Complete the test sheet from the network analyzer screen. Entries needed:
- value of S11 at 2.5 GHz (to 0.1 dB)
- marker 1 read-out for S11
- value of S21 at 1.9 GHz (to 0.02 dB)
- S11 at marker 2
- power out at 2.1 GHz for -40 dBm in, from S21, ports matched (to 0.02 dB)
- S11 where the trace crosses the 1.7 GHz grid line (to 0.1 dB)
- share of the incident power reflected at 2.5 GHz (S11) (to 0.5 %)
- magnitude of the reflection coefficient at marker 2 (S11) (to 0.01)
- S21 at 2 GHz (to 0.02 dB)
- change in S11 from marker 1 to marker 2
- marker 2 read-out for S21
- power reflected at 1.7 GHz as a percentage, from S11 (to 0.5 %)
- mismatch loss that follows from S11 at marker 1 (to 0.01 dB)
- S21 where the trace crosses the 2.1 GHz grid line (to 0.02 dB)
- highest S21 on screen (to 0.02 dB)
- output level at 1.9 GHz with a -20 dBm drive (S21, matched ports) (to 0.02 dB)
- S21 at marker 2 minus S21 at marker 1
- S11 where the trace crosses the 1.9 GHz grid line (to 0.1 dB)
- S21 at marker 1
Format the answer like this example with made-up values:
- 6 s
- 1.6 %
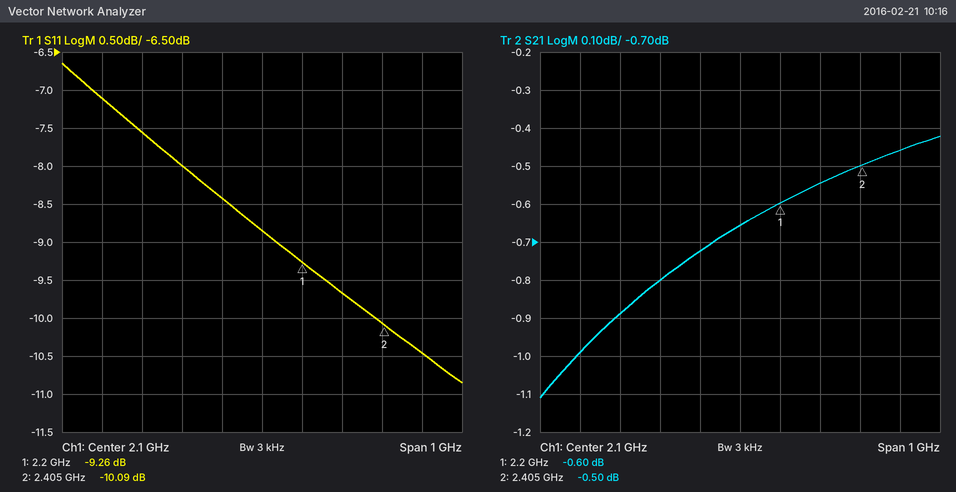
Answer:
- -10.5 dB
- -9.26 dB
- -0.80 dB
- -10.09 dB
- -40.66 dBm
- -7.1 dB
- 9.0 %
- 0.31
- -0.72 dB
- -0.83 dB
- -0.50 dB
- 19.5 %
- 0.55 dB
- -0.66 dB
- -0.42 dB
- -20.80 dBm
- 0.10 dB
- -8.0 dB
- -0.60 dB
